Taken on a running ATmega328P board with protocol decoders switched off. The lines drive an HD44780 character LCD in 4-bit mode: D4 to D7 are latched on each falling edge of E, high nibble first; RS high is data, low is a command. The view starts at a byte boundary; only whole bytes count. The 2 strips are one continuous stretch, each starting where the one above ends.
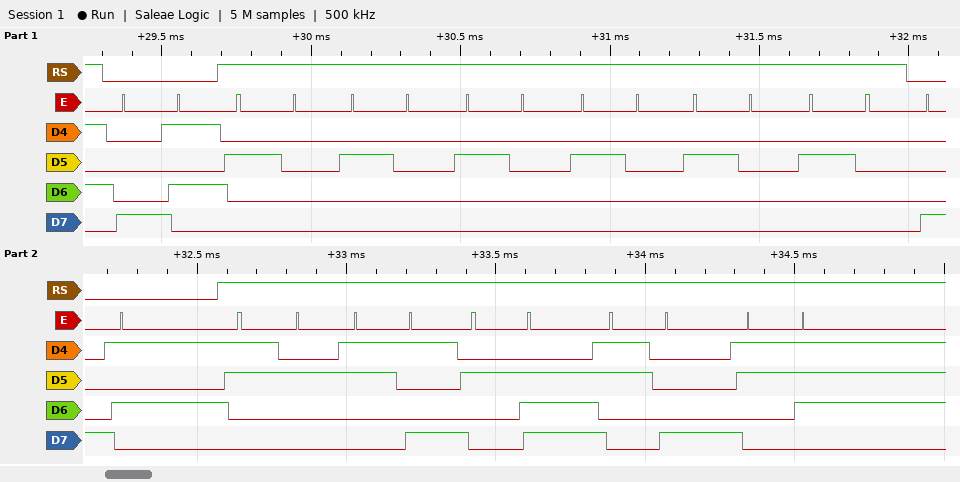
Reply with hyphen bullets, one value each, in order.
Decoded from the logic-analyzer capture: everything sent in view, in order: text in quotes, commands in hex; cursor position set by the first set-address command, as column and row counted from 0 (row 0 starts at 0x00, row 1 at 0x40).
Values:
- 0x85 "      " 0x85 "29.87"
- column 5, row 0
